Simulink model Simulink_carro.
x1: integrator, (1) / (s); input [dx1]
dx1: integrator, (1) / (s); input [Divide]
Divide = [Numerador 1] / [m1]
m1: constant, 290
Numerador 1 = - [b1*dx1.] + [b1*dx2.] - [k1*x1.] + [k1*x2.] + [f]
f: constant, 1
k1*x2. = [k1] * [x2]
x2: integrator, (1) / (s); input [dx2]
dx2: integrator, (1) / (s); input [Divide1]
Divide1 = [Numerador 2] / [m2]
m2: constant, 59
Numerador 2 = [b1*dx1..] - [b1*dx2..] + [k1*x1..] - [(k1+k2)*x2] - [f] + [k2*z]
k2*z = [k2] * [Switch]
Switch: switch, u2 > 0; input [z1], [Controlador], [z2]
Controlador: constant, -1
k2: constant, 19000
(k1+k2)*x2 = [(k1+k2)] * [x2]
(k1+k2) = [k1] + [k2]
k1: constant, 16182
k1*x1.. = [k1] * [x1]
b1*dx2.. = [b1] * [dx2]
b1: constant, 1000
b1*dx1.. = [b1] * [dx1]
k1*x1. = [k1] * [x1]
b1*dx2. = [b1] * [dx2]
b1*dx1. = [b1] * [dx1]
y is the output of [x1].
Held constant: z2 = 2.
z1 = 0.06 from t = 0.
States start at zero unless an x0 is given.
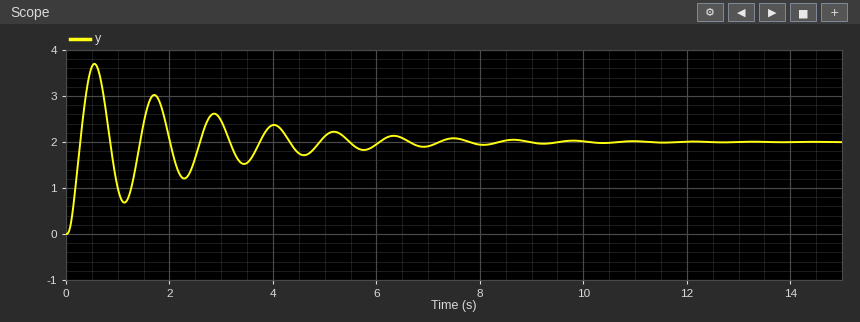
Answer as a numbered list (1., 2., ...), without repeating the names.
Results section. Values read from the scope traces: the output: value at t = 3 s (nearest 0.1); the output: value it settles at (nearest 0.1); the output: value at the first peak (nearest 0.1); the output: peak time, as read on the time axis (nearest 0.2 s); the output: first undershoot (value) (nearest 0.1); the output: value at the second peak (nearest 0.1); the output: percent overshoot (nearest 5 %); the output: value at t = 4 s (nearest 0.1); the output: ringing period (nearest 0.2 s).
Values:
1. 2.5
2. 2.0
3. 3.7
4. 0.6 s
5. 0.7
6. 3.0
7. 85 %
8. 2.4
9. 1.2 s
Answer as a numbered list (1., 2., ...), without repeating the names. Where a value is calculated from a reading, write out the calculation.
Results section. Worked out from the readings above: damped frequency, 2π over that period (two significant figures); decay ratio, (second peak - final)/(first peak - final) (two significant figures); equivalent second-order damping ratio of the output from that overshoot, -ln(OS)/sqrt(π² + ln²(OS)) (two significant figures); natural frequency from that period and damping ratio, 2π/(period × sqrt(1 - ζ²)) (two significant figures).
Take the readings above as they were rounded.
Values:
1. 2π / 1.2 = 5.2 rad/s
2. (3 - 2) / (3.7 - 2) = 0.59
3. ln(0.85) = -0.163; 0.163 / sqrt(9.870 + 0.026) = 0.052
4. 2π / (1.2 × sqrt(1 - 0.052²)) = 5.2 rad/s
